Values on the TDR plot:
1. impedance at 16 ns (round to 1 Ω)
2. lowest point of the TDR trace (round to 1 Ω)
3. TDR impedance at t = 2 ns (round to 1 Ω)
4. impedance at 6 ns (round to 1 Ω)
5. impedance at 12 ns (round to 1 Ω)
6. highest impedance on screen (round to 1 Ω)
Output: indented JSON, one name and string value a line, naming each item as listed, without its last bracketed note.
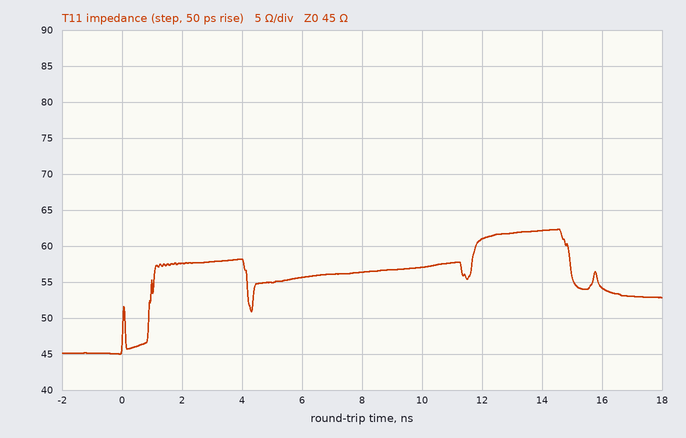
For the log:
{
  "impedance at 16 ns": "54 Ω",
  "lowest point of the TDR trace": "45 Ω",
  "TDR impedance at t = 2 ns": "58 Ω",
  "impedance at 6 ns": "56 Ω",
  "impedance at 12 ns": "61 Ω",
  "highest impedance on screen": "62 Ω"
}
